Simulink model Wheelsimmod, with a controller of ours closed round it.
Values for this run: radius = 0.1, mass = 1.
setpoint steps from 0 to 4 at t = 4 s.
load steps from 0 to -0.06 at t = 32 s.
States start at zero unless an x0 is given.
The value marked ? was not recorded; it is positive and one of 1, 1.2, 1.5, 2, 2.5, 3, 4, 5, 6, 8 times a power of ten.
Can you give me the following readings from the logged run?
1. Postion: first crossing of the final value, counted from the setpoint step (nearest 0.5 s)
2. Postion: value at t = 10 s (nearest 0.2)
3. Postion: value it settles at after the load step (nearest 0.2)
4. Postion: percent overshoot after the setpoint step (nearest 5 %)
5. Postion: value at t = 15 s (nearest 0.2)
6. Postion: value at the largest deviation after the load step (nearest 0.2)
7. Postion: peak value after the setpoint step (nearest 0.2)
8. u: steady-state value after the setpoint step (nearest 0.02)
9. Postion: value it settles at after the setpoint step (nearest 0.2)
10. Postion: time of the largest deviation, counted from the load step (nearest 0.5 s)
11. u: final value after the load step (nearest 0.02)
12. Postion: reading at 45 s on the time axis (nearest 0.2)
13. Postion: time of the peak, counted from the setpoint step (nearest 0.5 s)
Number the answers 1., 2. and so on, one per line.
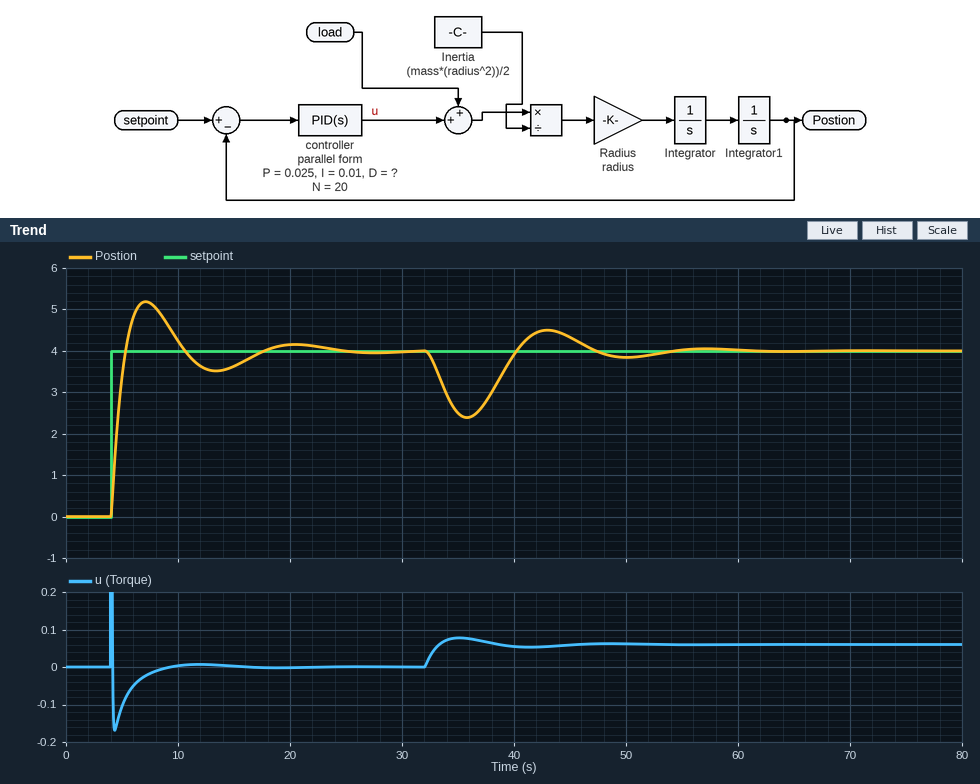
1. 1.5 s
2. 4.2
3. 4.0
4. 30 %
5. 3.6
6. 2.4
7. 5.2
8. 0.00
9. 4.0
10. 4.0 s
11. 0.06
12. 4.4
13. 3.0 s
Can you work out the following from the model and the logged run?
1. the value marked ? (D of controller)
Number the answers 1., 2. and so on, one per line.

1. 0.06
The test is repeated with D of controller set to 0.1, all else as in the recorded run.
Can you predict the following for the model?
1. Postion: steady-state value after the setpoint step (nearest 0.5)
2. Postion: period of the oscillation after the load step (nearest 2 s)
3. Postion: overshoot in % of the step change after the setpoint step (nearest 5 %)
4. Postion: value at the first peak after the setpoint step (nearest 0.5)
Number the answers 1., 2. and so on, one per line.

1. 4.0
2. 20 s
3. 15 %
4. 4.5
